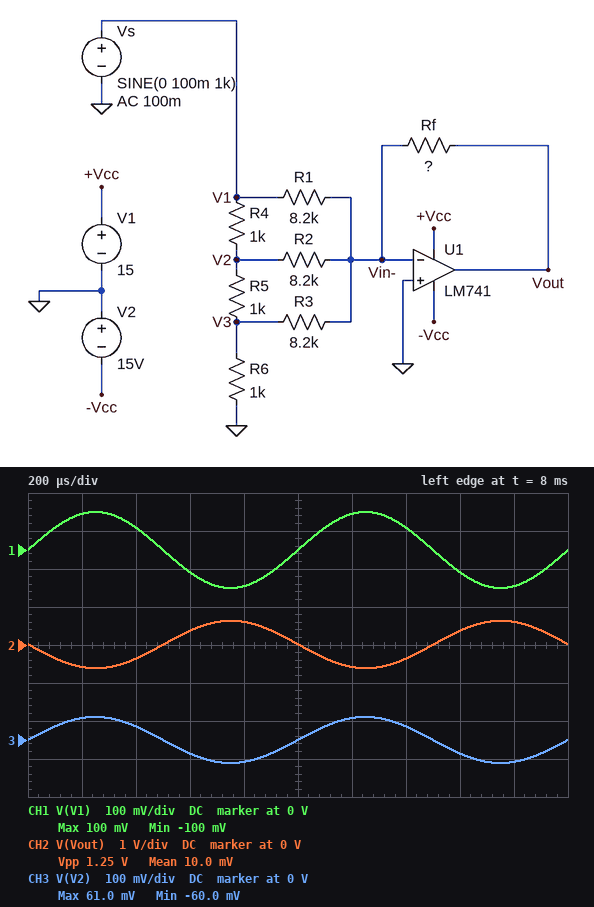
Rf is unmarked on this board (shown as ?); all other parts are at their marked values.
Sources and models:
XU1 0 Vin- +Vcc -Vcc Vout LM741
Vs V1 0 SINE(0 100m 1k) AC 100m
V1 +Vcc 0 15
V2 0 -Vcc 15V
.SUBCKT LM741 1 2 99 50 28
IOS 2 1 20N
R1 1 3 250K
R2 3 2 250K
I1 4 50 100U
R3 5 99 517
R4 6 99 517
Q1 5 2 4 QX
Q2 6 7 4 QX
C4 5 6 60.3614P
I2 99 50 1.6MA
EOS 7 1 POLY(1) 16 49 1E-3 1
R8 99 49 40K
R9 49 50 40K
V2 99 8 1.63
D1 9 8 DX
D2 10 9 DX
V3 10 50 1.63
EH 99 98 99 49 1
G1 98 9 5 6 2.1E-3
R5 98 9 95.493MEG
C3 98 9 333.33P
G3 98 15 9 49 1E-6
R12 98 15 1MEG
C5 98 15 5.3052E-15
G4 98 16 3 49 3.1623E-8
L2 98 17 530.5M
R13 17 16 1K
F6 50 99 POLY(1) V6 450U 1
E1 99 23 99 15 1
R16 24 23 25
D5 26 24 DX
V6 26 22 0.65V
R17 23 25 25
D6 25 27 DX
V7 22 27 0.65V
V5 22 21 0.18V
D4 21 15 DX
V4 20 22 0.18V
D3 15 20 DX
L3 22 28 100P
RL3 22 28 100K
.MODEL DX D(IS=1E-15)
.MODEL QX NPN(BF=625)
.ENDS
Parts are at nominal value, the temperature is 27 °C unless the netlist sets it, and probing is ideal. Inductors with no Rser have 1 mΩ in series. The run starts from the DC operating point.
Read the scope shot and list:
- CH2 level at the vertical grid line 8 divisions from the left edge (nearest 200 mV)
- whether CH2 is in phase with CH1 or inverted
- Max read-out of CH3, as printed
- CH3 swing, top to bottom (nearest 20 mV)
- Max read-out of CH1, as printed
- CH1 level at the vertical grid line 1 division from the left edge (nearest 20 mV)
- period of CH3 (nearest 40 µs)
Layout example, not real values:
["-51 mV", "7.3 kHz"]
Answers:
["400 mV", "inverted", "61.0 mV", "120 mV", "100 mV", "100 mV", "1.00 ms"]
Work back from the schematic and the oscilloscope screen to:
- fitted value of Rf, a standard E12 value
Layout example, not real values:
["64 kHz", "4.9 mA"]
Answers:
["27 kΩ"]
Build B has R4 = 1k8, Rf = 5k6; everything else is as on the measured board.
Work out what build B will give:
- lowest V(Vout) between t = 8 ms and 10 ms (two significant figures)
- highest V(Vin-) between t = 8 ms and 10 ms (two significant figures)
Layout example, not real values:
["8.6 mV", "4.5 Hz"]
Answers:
["-110 mV", "1.1 mV"]
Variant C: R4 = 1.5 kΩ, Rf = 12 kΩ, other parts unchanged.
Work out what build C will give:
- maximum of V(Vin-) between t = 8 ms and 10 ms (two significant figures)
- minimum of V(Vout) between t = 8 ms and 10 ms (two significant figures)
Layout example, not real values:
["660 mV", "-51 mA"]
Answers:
["1.3 mV", "-250 mV"]
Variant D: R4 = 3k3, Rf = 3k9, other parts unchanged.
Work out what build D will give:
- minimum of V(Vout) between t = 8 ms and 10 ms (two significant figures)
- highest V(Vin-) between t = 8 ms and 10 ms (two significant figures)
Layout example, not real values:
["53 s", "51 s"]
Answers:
["-67 mV", "1.1 mV"]
